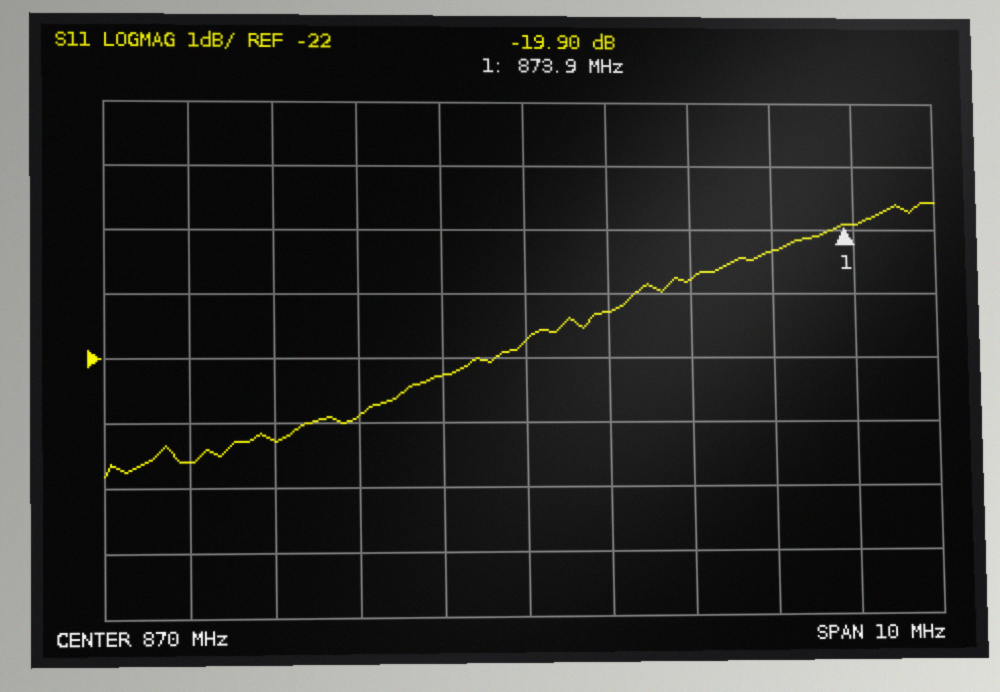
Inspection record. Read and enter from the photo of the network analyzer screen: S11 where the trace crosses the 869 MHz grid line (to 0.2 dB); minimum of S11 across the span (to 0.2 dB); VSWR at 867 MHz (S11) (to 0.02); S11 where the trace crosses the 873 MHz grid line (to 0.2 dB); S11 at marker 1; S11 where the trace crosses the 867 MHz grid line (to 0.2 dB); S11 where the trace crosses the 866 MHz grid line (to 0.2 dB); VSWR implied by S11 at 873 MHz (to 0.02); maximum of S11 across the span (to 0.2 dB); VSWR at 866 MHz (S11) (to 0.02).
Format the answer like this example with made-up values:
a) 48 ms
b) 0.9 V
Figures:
a) -22.2 dB
b) -23.8 dB
c) 1.14
d) -20.4 dB
e) -19.90 dB
f) -23.2 dB
g) -23.6 dB
h) 1.22
i) -19.6 dB
j) 1.14
